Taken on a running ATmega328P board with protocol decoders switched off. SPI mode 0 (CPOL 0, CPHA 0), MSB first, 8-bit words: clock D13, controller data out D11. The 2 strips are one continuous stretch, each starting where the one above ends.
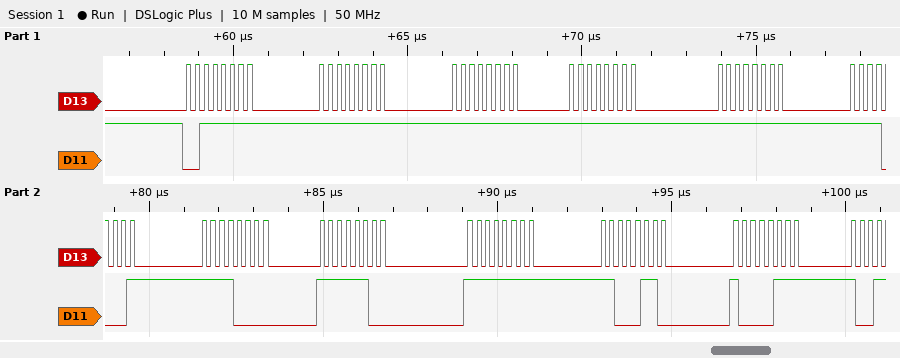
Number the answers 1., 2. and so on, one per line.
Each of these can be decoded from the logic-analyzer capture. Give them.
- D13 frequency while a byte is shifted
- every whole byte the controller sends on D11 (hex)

1. 4 MHz
2. 0x3F 0xFF 0xFF 0xFF 0xFF 0xF1 0xF0 0xFC 0xFF 0xC6 0x87
